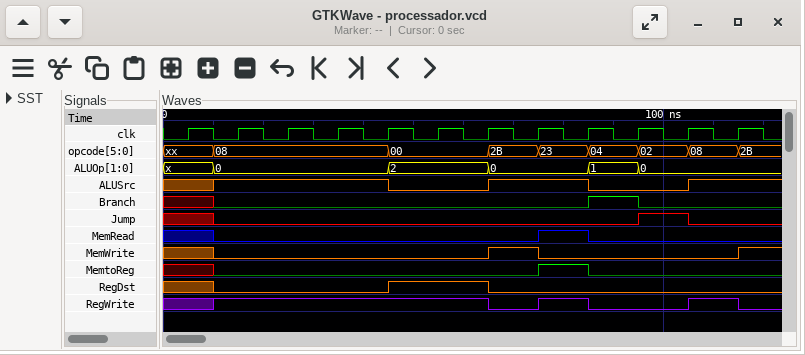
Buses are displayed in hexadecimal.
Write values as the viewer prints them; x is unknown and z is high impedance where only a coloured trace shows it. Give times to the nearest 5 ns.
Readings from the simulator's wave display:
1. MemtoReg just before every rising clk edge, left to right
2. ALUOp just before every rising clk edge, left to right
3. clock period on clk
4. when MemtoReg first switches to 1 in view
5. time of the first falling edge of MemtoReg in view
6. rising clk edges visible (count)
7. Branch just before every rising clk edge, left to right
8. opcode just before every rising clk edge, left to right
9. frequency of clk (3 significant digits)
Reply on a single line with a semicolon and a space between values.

x 0 0 0 0 0 0 0 1 0 0 0; x, 0, 0, 0, 0, 2, 2, 0, 0, 1, 0, 0; 10 ns; 75 ns; 85 ns; 12; x 0 0 0 0 0 0 0 0 1 0 0; xx, 08, 08, 08, 08, 00, 00, 2B, 23, 04, 02, 08; 100 MHz
